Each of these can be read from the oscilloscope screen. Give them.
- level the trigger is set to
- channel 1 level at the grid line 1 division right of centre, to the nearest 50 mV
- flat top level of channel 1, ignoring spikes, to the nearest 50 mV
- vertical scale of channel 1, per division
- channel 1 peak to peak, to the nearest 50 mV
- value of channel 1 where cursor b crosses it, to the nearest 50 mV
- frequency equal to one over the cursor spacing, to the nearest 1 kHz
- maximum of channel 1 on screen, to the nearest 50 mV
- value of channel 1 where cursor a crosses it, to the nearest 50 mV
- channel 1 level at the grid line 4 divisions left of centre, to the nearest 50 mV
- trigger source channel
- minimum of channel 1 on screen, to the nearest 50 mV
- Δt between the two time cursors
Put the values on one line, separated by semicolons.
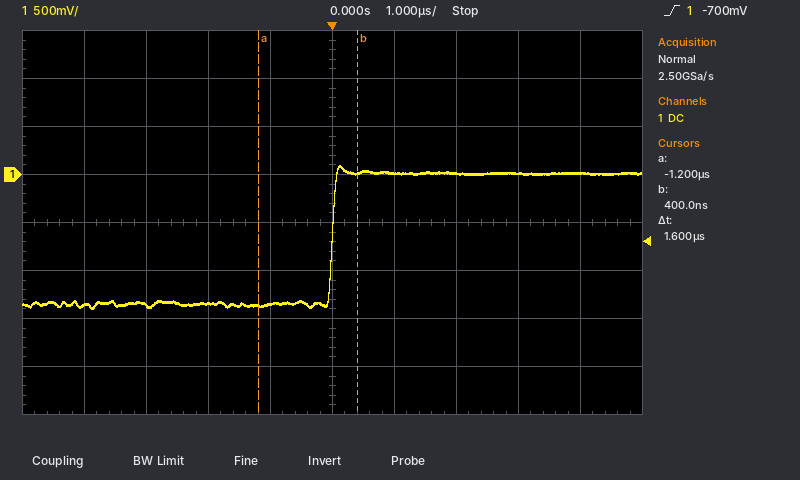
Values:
-700 mV; 0 mV; 0 mV; 500 mV; 1.50 V; 0 mV; 625 kHz; 100 mV; -1.35 V; -1.35 V; channel 1; -1.40 V; 1.6 µs
